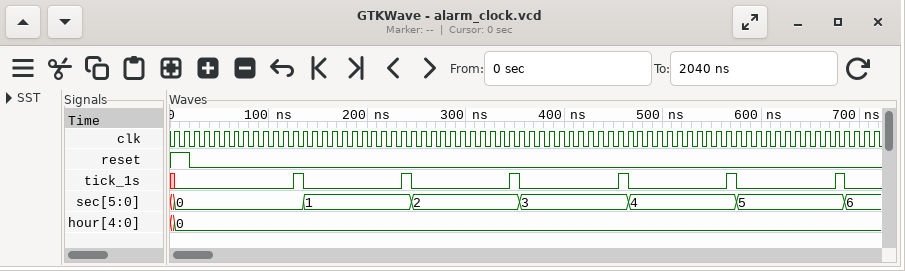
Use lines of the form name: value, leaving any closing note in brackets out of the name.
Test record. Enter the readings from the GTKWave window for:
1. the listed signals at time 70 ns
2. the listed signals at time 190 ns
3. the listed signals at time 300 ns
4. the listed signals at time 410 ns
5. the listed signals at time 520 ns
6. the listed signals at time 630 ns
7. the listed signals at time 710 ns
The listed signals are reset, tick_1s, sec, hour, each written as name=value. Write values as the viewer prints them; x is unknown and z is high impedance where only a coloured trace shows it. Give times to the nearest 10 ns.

the listed signals at time 70 ns: reset=0, tick_1s=0, sec=0, hour=0
the listed signals at time 190 ns: reset=0, tick_1s=0, sec=1, hour=0
the listed signals at time 300 ns: reset=0, tick_1s=0, sec=2, hour=0
the listed signals at time 410 ns: reset=0, tick_1s=0, sec=3, hour=0
the listed signals at time 520 ns: reset=0, tick_1s=0, sec=4, hour=0
the listed signals at time 630 ns: reset=0, tick_1s=0, sec=5, hour=0
the listed signals at time 710 ns: reset=0, tick_1s=0, sec=6, hour=0
